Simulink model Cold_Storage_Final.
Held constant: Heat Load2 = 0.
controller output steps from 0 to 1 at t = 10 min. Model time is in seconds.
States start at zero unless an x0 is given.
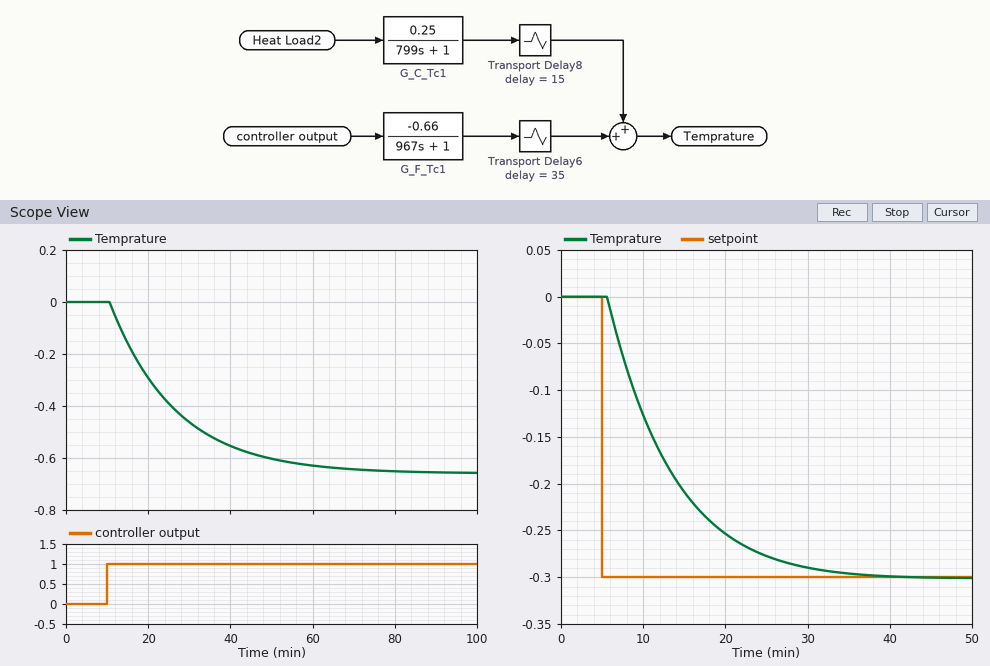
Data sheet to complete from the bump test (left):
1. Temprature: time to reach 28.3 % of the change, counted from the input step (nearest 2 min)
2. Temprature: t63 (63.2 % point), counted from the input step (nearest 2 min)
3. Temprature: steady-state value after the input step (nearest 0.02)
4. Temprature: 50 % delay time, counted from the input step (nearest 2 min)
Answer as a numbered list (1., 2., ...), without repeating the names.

1. 6 min
2. 16 min
3. -0.66
4. 12 min
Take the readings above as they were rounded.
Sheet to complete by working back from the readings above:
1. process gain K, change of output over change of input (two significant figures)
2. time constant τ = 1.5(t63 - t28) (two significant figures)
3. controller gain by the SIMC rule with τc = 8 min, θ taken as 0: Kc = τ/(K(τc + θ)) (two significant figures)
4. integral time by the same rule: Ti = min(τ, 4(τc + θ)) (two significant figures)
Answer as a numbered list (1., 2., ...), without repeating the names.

1. -0.66
2. 15 min
3. -2.8
4. 15 min
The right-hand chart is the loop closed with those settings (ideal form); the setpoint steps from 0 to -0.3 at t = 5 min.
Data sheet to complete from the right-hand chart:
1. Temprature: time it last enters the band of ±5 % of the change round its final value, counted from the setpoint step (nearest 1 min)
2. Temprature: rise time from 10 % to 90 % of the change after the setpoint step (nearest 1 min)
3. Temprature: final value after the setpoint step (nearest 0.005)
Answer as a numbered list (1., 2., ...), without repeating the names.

1. 23 min
2. 17 min
3. -0.300
